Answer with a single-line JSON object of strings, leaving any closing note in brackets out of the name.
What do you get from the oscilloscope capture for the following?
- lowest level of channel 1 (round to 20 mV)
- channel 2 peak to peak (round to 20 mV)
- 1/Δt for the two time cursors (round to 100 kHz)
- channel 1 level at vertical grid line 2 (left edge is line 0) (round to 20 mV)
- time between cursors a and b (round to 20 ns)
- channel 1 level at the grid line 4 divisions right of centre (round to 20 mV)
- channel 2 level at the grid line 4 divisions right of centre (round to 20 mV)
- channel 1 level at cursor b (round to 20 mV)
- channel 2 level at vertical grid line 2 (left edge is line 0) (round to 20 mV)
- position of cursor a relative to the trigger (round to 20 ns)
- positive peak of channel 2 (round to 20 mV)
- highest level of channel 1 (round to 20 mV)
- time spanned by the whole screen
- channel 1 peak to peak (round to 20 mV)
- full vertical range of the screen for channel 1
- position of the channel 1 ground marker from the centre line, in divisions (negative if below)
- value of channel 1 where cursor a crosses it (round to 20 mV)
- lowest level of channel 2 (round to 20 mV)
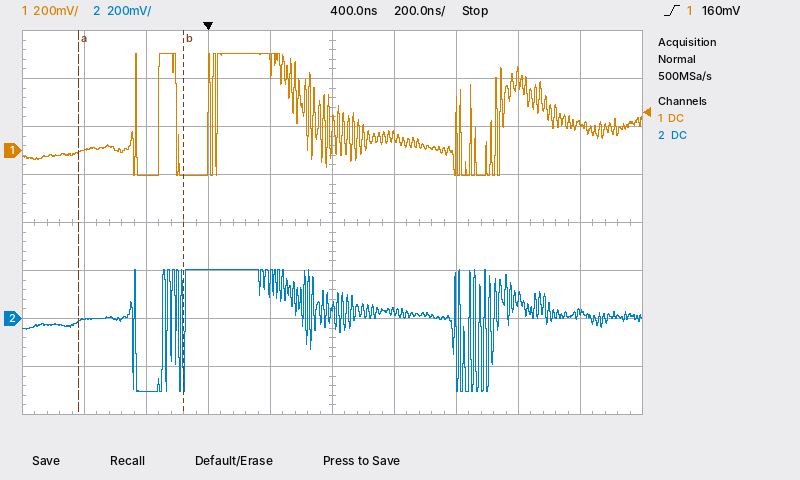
{"lowest level of channel 1": "-100 mV", "channel 2 peak to peak": "500 mV", "1/Δt for the two time cursors": "2.9 MHz", "channel 1 level at vertical grid line 2 (left edge is line 0)": "-100 mV", "time between cursors a and b": "340 ns", "channel 1 level at the grid line 4 divisions right of centre": "120 mV", "channel 2 level at the grid line 4 divisions right of centre": "20 mV", "channel 1 level at cursor b": "-100 mV", "channel 2 level at vertical grid line 2 (left edge is line 0)": "-300 mV", "position of cursor a relative to the trigger": "-420 ns", "positive peak of channel 2": "200 mV", "highest level of channel 1": "400 mV", "time spanned by the whole screen": "2 µs", "channel 1 peak to peak": "500 mV", "full vertical range of the screen for channel 1": "1.6 V", "position of the channel 1 ground marker from the centre line, in divisions": "+1.5 div", "value of channel 1 where cursor a crosses it": "0 mV", "lowest level of channel 2": "-300 mV"}
